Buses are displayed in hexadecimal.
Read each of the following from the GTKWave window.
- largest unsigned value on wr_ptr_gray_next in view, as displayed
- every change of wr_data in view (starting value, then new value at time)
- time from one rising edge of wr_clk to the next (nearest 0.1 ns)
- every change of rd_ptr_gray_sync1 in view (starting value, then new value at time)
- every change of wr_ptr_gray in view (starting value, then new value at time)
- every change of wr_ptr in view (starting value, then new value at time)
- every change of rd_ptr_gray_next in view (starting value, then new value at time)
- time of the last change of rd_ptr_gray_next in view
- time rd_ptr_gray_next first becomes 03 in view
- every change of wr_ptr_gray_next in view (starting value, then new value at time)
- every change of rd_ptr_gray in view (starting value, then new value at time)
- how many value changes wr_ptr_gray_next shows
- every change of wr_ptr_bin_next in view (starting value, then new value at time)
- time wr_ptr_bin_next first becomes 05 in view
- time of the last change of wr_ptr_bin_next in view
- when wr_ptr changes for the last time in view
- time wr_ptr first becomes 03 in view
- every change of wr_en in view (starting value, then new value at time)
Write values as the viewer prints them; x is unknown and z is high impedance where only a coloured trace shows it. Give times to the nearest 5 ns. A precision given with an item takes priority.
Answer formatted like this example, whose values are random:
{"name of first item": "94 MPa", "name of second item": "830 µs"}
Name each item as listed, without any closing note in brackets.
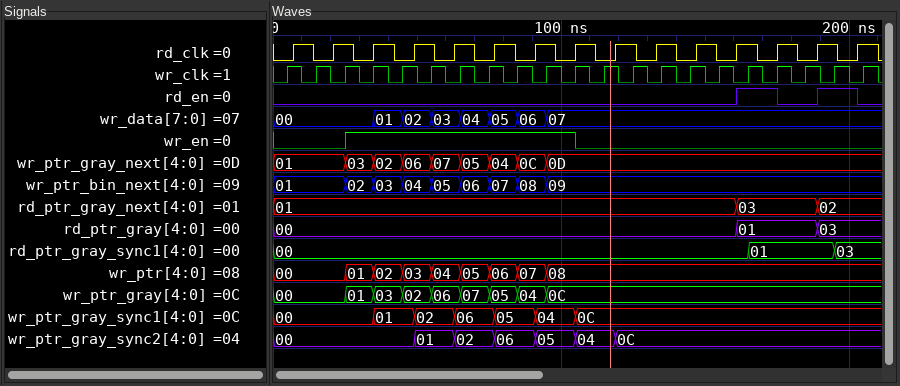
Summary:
{"largest unsigned value on wr_ptr_gray_next in view, as displayed": "0D", "every change of wr_data in view": "00, 01 at 35 ns, 02 at 45 ns, 03 at 55 ns, 04 at 65 ns, 05 at 75 ns, 06 at 85 ns, 07 at 95 ns", "time from one rising edge of wr_clk to the next": "10 ns", "every change of rd_ptr_gray_sync1 in view": "00, 01 at 165 ns, 03 at 195 ns", "every change of wr_ptr_gray in view": "00, 01 at 25 ns, 03 at 35 ns, 02 at 45 ns, 06 at 55 ns, 07 at 65 ns, 05 at 75 ns, 04 at 85 ns, 0C at 95 ns", "every change of wr_ptr in view": "00, 01 at 25 ns, 02 at 35 ns, 03 at 45 ns, 04 at 55 ns, 05 at 65 ns, 06 at 75 ns, 07 at 85 ns, 08 at 95 ns", "every change of rd_ptr_gray_next in view": "01, 03 at 160 ns, 02 at 190 ns", "time of the last change of rd_ptr_gray_next in view": "190 ns", "time rd_ptr_gray_next first becomes 03 in view": "160 ns", "every change of wr_ptr_gray_next in view": "01, 03 at 25 ns, 02 at 35 ns, 06 at 45 ns, 07 at 55 ns, 05 at 65 ns, 04 at 75 ns, 0C at 85 ns, 0D at 95 ns", "every change of rd_ptr_gray in view": "00, 01 at 160 ns, 03 at 190 ns", "how many value changes wr_ptr_gray_next shows": "8", "every change of wr_ptr_bin_next in view": "01, 02 at 25 ns, 03 at 35 ns, 04 at 45 ns, 05 at 55 ns, 06 at 65 ns, 07 at 75 ns, 08 at 85 ns, 09 at 95 ns", "time wr_ptr_bin_next first becomes 05 in view": "55 ns", "time of the last change of wr_ptr_bin_next in view": "95 ns", "when wr_ptr changes for the last time in view": "95 ns", "time wr_ptr first becomes 03 in view": "45 ns", "every change of wr_en in view": "0, 1 at 25 ns, 0 at 105 ns"}
